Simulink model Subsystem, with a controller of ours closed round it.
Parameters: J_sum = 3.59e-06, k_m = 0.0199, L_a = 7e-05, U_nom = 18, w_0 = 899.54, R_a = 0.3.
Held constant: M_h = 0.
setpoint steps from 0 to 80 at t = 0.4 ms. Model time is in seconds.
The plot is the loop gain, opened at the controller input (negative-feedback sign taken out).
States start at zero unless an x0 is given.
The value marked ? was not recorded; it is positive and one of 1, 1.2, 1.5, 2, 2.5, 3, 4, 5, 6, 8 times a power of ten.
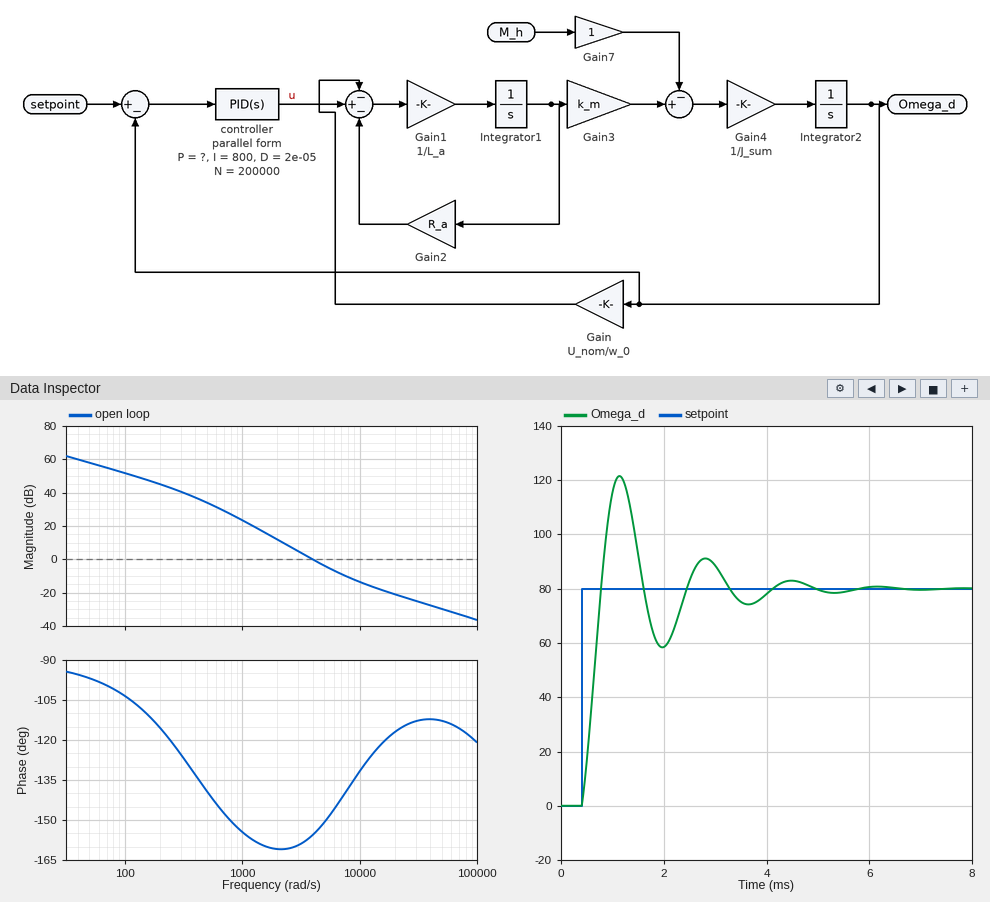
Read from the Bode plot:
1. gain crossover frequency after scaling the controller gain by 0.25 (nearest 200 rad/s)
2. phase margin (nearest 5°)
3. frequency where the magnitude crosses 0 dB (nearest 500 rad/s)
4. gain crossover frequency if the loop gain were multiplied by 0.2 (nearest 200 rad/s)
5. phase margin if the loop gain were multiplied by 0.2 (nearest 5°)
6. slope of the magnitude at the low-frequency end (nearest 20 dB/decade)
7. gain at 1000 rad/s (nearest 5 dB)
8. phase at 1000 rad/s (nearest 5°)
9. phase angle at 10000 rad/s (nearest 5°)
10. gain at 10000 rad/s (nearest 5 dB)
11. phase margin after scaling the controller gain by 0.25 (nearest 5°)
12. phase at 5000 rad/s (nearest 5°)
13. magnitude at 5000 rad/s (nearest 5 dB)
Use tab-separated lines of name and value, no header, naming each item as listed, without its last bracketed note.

gain crossover frequency after scaling the controller gain by 0.25	2000 rad/s
phase margin	25°
frequency where the magnitude crosses 0 dB	4000 rad/s
gain crossover frequency if the loop gain were multiplied by 0.2	1800 rad/s
phase margin if the loop gain were multiplied by 0.2	20°
slope of the magnitude at the low-frequency end	-20 dB/decade
gain at 1000 rad/s	25 dB
phase at 1000 rad/s	-155°
phase angle at 10000 rad/s	-130°
gain at 10000 rad/s	-15 dB
phase margin after scaling the controller gain by 0.25	20°
phase at 5000 rad/s	-150°
magnitude at 5000 rad/s	-5 dB
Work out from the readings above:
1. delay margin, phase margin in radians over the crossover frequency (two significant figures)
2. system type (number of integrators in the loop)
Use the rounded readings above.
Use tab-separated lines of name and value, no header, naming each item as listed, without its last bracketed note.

delay margin, phase margin in radians over the crossover frequency	0.00011 s
system type	1
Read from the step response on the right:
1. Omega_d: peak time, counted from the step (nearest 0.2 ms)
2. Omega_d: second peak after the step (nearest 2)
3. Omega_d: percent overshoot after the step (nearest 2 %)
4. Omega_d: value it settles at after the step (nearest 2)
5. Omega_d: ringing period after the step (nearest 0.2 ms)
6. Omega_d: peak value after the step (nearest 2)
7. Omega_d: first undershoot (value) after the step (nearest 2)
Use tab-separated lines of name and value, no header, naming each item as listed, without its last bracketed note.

Omega_d: peak time, counted from the step	0.8 ms
Omega_d: second peak after the step	92
Omega_d: percent overshoot after the step	52 %
Omega_d: value it settles at after the step	80
Omega_d: ringing period after the step	1.6 ms
Omega_d: peak value after the step	122
Omega_d: first undershoot (value) after the step	58
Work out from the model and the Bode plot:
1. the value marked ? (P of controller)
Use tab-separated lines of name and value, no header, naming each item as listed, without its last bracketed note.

the value marked ?	0.25
